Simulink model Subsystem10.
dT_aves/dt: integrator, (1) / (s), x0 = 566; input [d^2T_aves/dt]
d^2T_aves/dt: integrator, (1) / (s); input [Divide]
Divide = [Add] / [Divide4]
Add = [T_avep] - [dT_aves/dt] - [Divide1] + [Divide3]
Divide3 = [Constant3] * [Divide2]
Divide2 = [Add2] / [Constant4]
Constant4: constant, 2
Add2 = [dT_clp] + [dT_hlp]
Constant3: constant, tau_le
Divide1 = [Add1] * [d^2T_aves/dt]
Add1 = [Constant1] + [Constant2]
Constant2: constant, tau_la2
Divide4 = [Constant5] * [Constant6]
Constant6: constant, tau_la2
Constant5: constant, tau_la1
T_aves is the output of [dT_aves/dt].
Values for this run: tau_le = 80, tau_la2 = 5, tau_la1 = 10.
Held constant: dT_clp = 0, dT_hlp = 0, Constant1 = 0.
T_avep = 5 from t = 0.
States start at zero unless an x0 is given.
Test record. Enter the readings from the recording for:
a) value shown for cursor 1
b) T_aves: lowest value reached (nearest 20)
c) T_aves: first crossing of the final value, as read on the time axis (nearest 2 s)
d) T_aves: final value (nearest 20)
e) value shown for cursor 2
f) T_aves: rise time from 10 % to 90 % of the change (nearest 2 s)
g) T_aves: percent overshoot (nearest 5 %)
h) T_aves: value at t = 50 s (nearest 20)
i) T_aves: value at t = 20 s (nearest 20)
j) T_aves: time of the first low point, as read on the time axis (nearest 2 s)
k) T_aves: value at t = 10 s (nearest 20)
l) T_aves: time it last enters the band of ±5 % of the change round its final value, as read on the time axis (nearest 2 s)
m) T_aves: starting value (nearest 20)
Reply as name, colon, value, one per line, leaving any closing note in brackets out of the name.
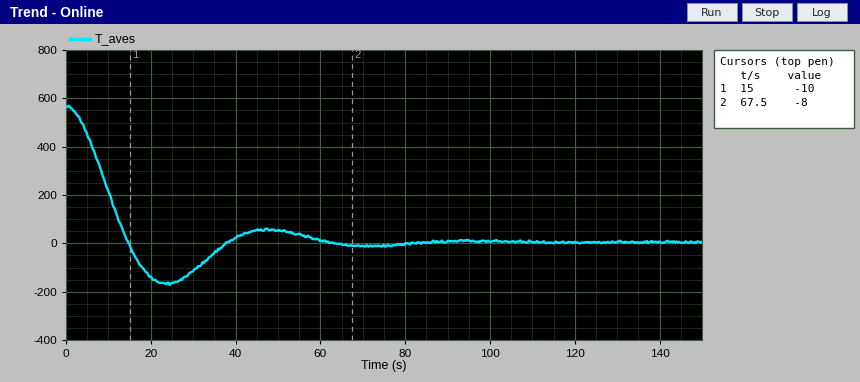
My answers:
value shown for cursor 1: -10
T_aves: lowest value reached: -160
T_aves: first crossing of the final value, as read on the time axis: 14 s
T_aves: final value: 0
value shown for cursor 2: -8
T_aves: rise time from 10 % to 90 % of the change: 10 s
T_aves: percent overshoot: 30 %
T_aves: value at t = 50 s: 60
T_aves: value at t = 20 s: -140
T_aves: time of the first low point, as read on the time axis: 24 s
T_aves: value at t = 10 s: 220
T_aves: time it last enters the band of ±5 % of the change round its final value, as read on the time axis: 56 s
T_aves: starting value: 560
